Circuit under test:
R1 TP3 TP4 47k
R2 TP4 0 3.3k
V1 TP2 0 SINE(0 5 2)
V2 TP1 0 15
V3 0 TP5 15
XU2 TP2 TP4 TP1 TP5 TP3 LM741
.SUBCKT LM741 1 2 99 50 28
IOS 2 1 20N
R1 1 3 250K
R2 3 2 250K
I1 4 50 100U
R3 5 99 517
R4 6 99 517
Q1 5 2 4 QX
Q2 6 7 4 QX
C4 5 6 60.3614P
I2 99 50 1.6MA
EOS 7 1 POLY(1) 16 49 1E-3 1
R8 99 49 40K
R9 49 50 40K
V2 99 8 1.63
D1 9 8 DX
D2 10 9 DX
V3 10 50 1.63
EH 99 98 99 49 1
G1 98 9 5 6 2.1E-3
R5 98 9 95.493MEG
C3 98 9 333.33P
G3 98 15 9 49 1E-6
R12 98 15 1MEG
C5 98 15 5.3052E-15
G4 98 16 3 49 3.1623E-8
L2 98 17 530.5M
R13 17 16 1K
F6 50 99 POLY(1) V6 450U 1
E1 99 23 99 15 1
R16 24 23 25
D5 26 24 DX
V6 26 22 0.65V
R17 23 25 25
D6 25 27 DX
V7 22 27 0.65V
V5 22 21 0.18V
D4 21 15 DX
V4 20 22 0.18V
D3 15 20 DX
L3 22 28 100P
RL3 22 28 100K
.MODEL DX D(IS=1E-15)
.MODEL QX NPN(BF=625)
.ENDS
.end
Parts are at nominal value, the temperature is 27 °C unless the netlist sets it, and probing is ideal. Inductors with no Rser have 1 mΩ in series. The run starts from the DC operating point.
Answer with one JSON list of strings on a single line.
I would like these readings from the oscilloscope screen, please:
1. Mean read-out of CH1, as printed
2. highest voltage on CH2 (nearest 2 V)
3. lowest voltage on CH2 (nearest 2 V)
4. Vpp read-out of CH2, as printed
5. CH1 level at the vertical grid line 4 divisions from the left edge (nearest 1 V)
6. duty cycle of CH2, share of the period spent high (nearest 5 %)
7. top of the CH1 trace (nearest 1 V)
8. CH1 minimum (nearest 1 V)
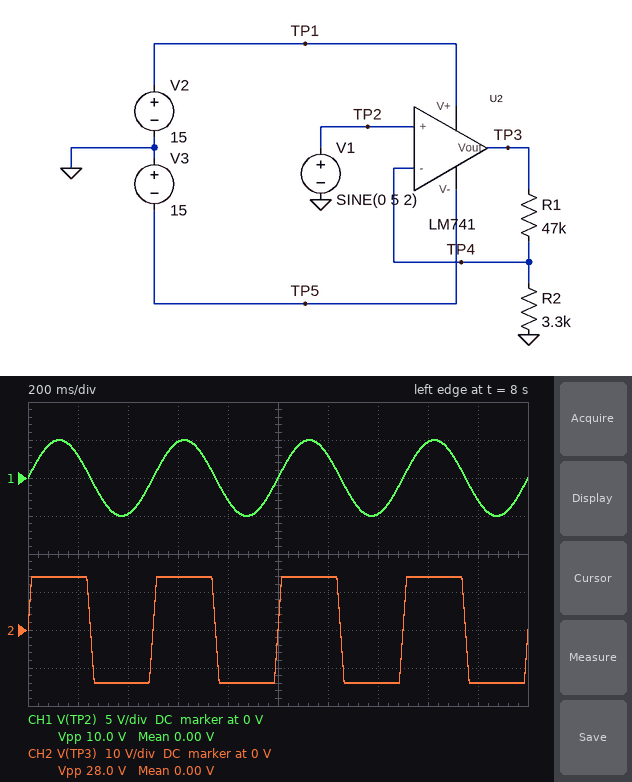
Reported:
["0.00 V", "14 V", "-14 V", "28.0 V", "-3 V", "50 %", "5 V", "-5 V"]
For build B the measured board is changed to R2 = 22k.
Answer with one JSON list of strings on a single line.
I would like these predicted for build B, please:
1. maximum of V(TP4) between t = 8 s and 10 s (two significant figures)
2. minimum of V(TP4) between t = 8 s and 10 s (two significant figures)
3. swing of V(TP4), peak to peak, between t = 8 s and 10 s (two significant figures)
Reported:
["4.5 V", "-4.5 V", "9.0 V"]
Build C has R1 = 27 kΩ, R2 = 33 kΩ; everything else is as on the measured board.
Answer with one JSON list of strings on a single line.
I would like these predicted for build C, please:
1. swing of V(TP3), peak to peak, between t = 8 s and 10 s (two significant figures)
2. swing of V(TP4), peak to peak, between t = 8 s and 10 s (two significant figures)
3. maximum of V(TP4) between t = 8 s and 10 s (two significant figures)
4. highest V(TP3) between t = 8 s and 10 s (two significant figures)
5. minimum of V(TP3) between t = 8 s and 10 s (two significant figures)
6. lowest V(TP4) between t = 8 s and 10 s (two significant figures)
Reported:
["18 V", "10 V", "5.0 V", "9.1 V", "-9.1 V", "-5.0 V"]
